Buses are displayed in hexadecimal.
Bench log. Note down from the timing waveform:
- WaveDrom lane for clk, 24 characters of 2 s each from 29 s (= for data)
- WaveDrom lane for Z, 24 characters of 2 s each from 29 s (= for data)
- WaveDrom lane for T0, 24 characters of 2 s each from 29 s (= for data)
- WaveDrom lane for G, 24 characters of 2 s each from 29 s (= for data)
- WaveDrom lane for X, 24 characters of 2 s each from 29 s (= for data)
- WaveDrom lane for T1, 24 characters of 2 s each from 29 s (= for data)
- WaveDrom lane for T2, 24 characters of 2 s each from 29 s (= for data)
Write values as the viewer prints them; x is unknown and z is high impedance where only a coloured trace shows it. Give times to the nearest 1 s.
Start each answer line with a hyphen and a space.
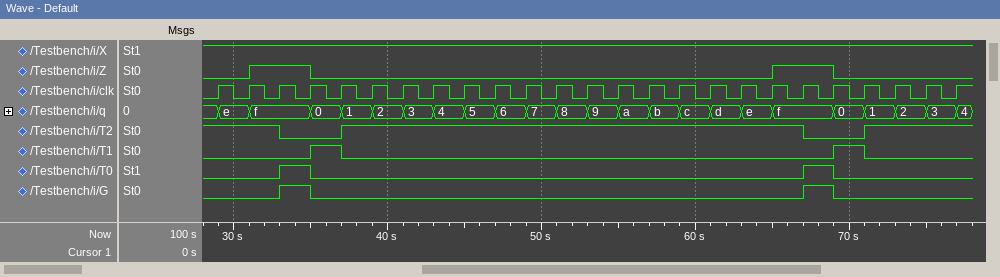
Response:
- {name: 'clk', wave: 'p.......................'}
- {name: 'Z', wave: '01.0..............1.0...'}
- {name: 'T0', wave: '0.10...............10...'}
- {name: 'G', wave: '0.10...............10...'}
- {name: 'X', wave: '1.......................'}
- {name: 'T1', wave: '0..10...............10..'}
- {name: 'T2', wave: '1.0.1..............0.1..'}
